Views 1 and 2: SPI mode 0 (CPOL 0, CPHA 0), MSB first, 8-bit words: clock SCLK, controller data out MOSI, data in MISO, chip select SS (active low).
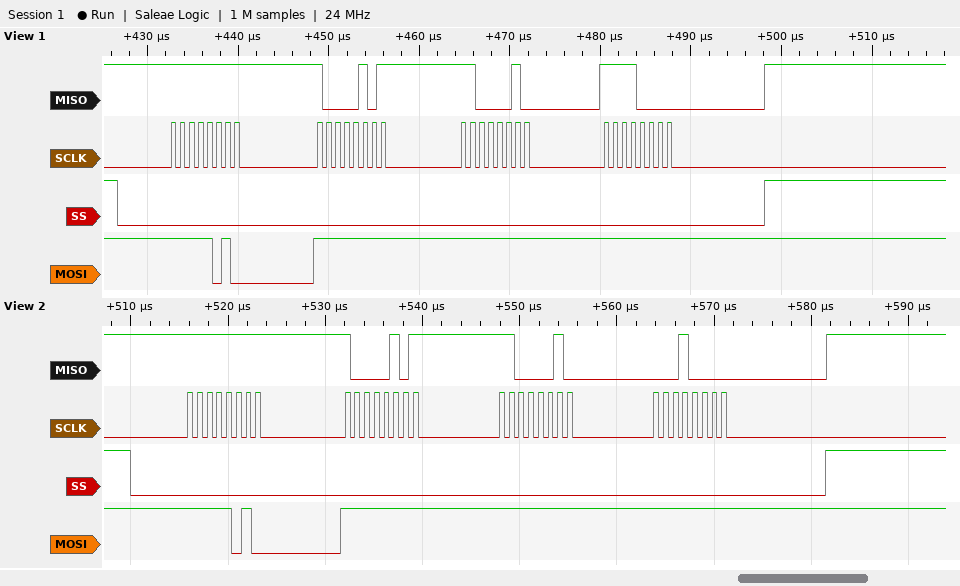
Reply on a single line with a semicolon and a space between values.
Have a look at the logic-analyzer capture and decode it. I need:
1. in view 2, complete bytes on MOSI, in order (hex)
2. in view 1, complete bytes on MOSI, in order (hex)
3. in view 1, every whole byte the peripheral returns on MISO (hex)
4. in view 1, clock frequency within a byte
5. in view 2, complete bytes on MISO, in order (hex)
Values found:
FA FF FF FF; FA FF FF FF; FF 85 C2 F0; 1 MHz; FF 85 C2 10
